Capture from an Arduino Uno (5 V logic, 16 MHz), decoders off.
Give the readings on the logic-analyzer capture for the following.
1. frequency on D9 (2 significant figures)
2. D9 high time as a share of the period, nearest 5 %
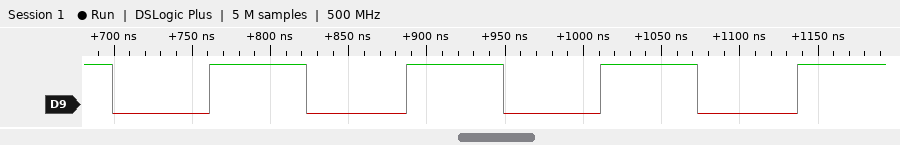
8.0 MHz
50 %
